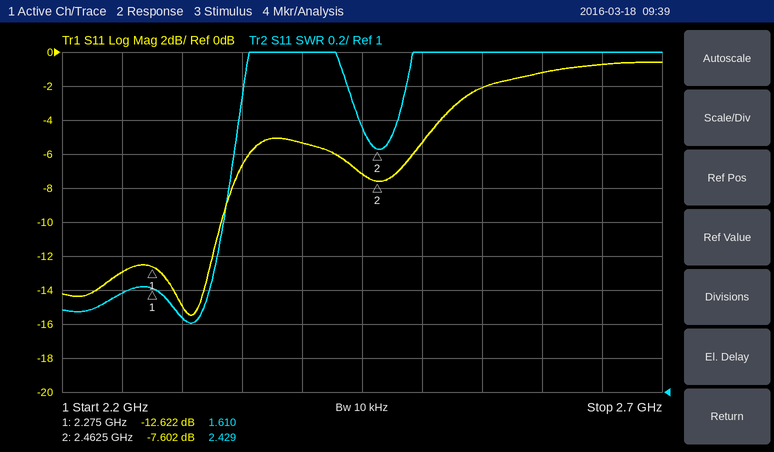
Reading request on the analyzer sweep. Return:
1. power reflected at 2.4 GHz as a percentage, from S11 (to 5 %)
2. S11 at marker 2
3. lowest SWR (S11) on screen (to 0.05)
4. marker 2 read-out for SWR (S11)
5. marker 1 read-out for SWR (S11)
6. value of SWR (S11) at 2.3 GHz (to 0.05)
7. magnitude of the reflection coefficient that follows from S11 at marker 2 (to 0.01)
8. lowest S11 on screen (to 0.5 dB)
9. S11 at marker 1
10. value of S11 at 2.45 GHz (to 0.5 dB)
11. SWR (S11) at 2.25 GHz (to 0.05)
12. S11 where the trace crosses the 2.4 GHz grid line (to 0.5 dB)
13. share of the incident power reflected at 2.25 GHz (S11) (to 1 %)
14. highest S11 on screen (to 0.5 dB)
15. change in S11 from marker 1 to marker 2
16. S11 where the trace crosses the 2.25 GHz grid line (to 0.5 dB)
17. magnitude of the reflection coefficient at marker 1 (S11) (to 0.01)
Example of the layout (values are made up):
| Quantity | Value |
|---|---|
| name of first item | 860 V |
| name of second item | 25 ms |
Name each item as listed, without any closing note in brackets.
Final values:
| Quantity | Value |
|---|---|
| power reflected at 2.4 GHz as a percentage, from S11 | 30 % |
| S11 at marker 2 | -7.602 dB |
| lowest SWR (S11) on screen | 1.40 |
| marker 2 read-out for SWR | 2.429 |
| marker 1 read-out for SWR | 1.610 |
| value of SWR (S11) at 2.3 GHz | 1.45 |
| magnitude of the reflection coefficient that follows from S11 at marker 2 | 0.42 |
| lowest S11 on screen | -15.5 dB |
| S11 at marker 1 | -12.622 dB |
| value of S11 at 2.45 GHz | -7.0 dB |
| SWR (S11) at 2.25 GHz | 1.60 |
| S11 where the trace crosses the 2.4 GHz grid line | -5.5 dB |
| share of the incident power reflected at 2.25 GHz (S11) | 5 % |
| highest S11 on screen | -0.5 dB |
| change in S11 from marker 1 to marker 2 | 5.020 dB |
| S11 where the trace crosses the 2.25 GHz grid line | -13.0 dB |
| magnitude of the reflection coefficient at marker 1 (S11) | 0.23 |
